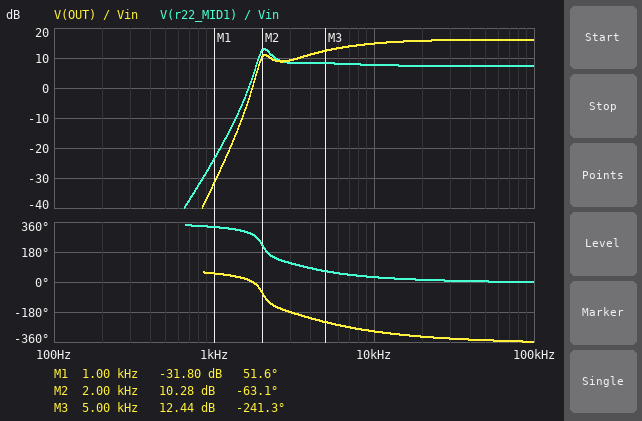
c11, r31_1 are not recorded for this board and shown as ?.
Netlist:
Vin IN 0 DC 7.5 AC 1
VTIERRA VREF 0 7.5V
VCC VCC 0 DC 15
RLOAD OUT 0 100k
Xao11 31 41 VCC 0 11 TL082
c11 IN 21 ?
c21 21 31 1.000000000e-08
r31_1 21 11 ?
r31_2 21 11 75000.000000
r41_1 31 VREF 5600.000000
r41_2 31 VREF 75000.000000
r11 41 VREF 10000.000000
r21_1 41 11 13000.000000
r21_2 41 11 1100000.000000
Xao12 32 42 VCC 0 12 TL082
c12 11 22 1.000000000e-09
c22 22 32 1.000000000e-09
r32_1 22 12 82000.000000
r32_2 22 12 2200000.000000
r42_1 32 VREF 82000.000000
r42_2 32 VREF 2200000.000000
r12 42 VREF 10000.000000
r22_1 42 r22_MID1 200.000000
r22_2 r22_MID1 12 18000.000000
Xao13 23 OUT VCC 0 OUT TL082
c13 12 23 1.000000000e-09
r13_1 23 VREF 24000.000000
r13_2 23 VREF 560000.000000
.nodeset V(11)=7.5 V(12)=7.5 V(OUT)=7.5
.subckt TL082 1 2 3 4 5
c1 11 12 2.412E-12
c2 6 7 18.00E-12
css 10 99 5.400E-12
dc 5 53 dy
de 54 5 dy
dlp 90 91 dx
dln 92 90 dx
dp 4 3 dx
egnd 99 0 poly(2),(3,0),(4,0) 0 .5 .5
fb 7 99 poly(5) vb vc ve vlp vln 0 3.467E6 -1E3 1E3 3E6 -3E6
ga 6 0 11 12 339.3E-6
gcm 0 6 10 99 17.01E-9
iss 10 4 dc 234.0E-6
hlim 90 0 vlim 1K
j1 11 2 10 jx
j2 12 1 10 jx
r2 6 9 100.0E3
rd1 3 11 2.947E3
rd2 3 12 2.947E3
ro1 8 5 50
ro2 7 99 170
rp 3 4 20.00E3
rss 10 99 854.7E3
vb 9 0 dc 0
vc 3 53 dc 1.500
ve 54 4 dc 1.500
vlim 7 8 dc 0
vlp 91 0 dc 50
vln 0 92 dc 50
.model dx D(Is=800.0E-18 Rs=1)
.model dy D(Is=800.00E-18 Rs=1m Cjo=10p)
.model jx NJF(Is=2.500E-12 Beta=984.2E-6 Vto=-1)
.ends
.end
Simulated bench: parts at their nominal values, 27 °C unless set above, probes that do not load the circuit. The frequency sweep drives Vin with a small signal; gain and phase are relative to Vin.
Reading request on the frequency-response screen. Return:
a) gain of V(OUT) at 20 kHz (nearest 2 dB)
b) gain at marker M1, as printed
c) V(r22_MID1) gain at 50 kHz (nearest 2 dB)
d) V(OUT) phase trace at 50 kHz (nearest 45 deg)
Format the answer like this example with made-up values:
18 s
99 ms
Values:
16 dB
-31.80 dB
8 dB
-360 deg
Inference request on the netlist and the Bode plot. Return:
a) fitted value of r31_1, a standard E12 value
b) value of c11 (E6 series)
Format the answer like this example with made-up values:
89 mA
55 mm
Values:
10 kΩ
4.7 nF
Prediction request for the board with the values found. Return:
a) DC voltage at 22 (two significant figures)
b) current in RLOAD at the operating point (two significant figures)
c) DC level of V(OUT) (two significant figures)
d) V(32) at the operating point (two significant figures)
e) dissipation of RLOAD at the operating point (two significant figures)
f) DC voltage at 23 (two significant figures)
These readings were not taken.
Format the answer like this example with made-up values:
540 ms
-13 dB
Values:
7.5 V
75 µA
7.5 V
7.5 V
560 µW
7.5 V
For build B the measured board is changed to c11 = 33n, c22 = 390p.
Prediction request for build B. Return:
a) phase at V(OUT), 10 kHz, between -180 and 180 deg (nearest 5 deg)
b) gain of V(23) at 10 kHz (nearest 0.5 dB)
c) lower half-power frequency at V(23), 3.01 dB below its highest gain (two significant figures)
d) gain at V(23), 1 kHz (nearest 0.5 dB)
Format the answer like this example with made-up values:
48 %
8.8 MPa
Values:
75 deg
14.5 dB
6.9 kHz
-31.0 dB
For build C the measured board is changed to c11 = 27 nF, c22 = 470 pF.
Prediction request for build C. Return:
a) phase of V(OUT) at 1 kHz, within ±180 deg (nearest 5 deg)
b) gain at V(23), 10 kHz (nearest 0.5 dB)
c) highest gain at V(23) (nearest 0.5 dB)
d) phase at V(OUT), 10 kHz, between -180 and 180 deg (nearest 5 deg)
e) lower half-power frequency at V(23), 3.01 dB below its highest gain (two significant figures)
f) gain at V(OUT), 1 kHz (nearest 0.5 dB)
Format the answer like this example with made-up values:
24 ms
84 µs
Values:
-10 deg
14.5 dB
16.0 dB
70 deg
6.4 kHz
-29.5 dB
